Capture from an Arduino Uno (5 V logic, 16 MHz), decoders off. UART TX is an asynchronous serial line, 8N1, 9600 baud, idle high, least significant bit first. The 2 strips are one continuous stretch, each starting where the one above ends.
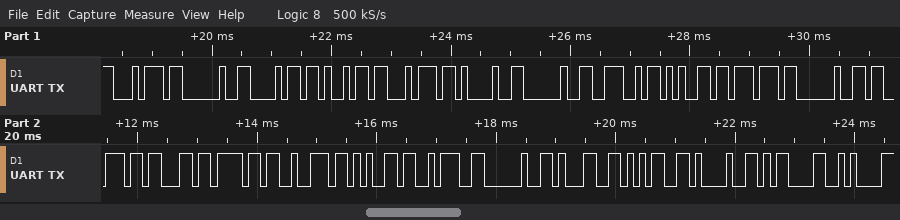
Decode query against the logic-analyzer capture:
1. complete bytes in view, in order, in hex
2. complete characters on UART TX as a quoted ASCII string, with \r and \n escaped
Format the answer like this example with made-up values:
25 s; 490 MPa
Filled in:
74 20 68 69 74 21 20 4E 65 77 20 73 63 6F 72 65 3A 20 31 35 21 0D 0A; "t hit! New score: 15!\r\n"
